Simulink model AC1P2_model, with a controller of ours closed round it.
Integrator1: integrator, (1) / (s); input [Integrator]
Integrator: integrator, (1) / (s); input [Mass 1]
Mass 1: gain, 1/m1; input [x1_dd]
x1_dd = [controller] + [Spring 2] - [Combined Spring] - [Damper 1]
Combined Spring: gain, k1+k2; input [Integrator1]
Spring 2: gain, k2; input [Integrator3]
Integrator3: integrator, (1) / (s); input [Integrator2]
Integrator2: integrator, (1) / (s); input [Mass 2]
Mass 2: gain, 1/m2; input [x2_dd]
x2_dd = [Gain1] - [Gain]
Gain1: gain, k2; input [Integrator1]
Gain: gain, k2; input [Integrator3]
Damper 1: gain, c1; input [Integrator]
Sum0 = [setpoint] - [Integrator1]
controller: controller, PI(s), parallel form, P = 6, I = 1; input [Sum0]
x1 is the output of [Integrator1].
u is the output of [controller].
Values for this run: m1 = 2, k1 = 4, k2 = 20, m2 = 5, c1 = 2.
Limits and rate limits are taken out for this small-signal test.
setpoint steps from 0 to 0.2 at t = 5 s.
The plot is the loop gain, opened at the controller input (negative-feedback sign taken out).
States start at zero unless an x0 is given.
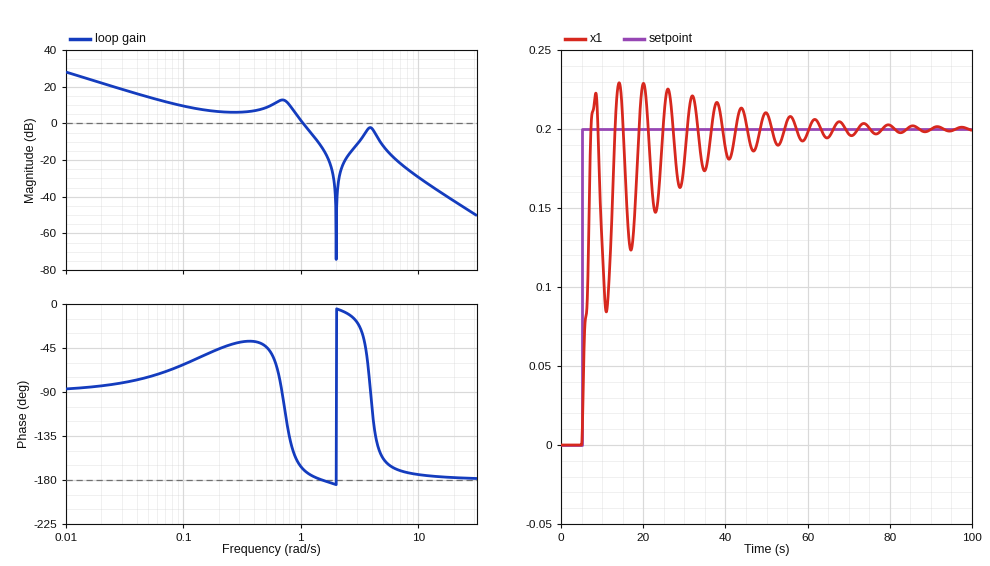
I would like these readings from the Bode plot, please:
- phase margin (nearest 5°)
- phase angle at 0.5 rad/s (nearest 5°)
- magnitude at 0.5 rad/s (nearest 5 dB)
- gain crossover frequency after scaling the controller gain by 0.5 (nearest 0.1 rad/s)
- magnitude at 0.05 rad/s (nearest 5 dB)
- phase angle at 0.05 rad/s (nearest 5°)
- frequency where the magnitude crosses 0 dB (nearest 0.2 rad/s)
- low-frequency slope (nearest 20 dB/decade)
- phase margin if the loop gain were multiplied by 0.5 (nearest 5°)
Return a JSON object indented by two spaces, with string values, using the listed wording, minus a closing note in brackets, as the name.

{
  "phase margin": "10°",
  "phase angle at 0.5 rad/s": "-45°",
  "magnitude at 0.5 rad/s": "10 dB",
  "gain crossover frequency after scaling the controller gain by 0.5": "0.9 rad/s",
  "magnitude at 0.05 rad/s": "15 dB",
  "phase angle at 0.05 rad/s": "-75°",
  "frequency where the magnitude crosses 0 dB": "1.0 rad/s",
  "low-frequency slope": "-20 dB/decade",
  "phase margin if the loop gain were multiplied by 0.5": "25°"
}
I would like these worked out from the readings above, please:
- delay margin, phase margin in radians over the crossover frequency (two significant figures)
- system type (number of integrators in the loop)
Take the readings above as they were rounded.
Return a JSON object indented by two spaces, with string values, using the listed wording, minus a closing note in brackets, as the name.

{
  "delay margin, phase margin in radians over the crossover frequency": "0.17 s",
  "system type": "1"
}
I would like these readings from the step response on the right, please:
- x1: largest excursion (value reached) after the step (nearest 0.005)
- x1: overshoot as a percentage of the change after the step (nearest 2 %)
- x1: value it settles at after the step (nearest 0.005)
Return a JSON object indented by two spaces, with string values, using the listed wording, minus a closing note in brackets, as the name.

{
  "x1: largest excursion (value reached) after the step": "0.230",
  "x1: overshoot as a percentage of the change after the step": "14 %",
  "x1: value it settles at after the step": "0.200"
}
